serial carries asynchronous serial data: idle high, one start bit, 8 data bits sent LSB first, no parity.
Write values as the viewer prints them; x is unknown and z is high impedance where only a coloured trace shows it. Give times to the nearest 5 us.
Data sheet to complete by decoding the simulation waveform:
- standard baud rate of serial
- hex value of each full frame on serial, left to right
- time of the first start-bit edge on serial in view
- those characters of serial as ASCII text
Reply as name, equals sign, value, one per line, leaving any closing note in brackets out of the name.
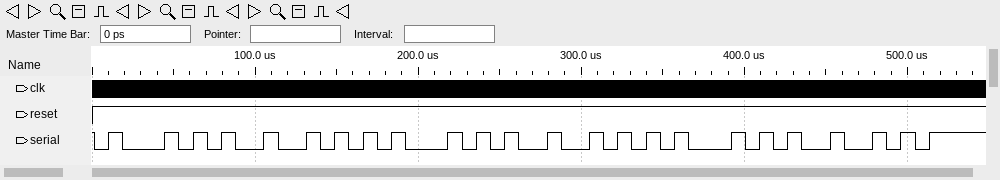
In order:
standard baud rate of serial = 115200 baud
hex value of each full frame on serial, left to right = 51, 52, 51, 52, 51, 52
time of the first start-bit edge on serial in view = 0 us
those characters of serial as ASCII text = "QRQRQR"
